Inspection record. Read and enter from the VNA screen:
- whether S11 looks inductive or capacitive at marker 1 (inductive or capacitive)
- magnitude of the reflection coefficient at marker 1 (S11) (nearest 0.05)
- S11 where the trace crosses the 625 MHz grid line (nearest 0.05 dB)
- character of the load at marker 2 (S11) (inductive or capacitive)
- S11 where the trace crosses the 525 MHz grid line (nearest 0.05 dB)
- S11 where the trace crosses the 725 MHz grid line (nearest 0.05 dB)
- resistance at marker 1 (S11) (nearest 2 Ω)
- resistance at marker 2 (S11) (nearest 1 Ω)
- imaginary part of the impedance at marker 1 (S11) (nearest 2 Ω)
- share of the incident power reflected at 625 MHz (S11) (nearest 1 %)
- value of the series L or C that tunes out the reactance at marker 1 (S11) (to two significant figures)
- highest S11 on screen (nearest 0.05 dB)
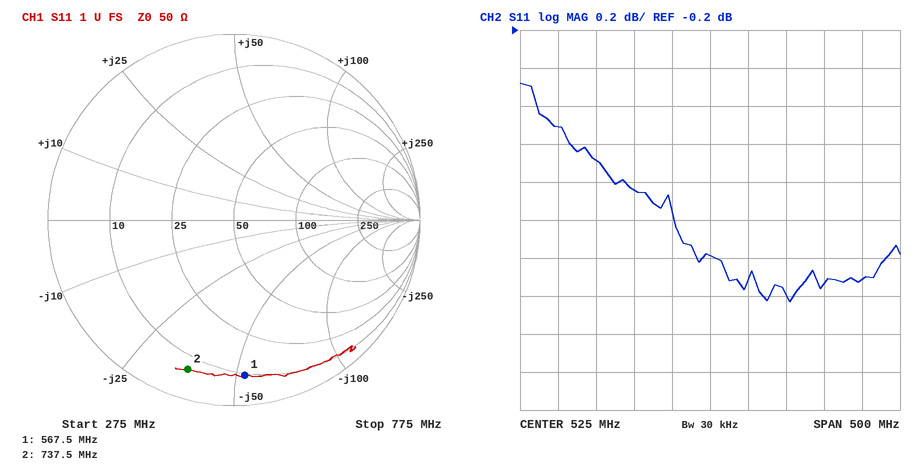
capacitive
0.85
-1.60 dB
capacitive
-1.40 dB
-1.50 dB
10 Ω
7 Ω
-52 Ω
69 %
15 nH
-0.50 dB
